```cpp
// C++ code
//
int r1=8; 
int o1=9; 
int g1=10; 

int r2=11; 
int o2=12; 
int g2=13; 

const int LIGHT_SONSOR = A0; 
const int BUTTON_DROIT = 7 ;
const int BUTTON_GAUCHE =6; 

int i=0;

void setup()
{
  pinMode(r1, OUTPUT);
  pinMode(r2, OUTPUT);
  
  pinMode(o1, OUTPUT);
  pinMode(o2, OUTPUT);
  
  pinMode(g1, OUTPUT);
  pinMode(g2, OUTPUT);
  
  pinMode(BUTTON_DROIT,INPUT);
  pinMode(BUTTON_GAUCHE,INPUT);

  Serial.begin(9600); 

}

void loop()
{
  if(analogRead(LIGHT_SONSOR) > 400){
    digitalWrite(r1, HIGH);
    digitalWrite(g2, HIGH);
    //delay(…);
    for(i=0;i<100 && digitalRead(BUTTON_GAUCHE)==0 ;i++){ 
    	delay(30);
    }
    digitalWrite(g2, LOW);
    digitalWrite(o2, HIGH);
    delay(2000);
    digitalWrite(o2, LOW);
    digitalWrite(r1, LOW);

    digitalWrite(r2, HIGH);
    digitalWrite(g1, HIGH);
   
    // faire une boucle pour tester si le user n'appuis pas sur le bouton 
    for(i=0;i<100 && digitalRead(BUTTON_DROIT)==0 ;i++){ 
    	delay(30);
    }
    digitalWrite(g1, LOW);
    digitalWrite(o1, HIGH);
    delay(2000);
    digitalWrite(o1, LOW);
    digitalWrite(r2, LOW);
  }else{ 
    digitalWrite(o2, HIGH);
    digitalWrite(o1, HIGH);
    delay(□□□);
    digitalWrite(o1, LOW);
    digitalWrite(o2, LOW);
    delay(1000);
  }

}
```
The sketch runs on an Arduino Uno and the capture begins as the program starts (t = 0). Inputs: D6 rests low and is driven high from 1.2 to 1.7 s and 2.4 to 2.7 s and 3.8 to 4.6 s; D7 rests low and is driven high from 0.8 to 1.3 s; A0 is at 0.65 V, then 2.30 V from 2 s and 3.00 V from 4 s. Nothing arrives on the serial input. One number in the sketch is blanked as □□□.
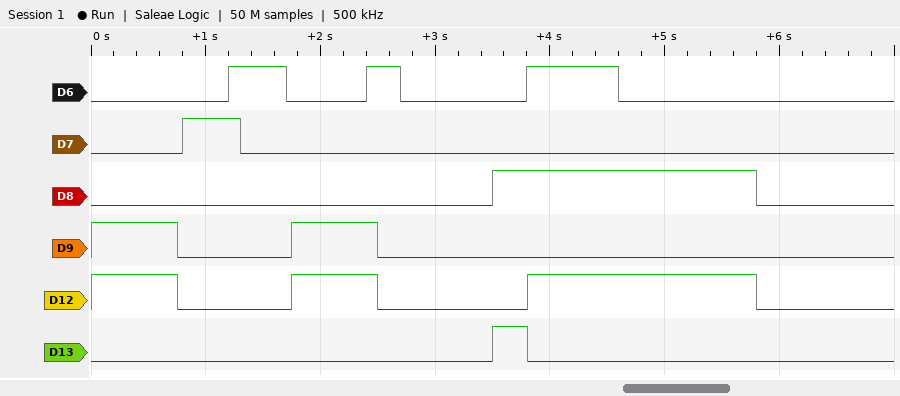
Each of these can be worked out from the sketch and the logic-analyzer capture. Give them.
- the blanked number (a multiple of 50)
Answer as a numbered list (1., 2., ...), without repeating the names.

1. 750
